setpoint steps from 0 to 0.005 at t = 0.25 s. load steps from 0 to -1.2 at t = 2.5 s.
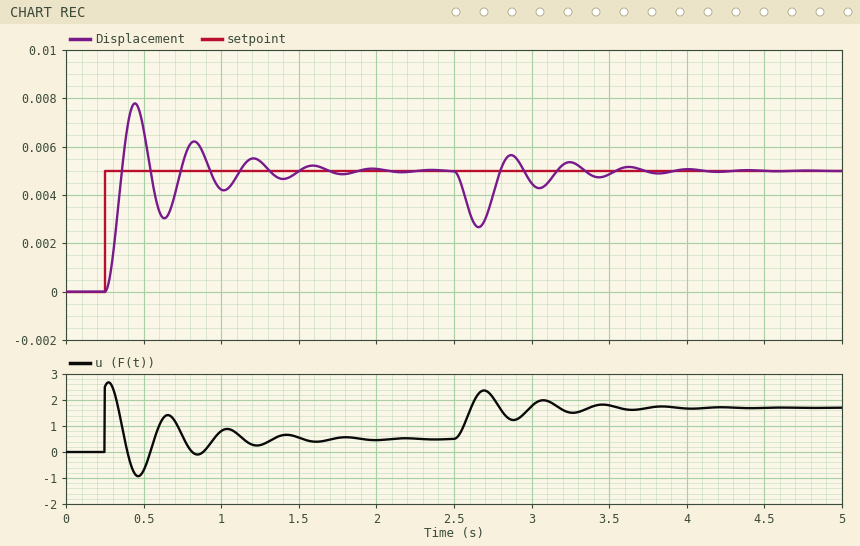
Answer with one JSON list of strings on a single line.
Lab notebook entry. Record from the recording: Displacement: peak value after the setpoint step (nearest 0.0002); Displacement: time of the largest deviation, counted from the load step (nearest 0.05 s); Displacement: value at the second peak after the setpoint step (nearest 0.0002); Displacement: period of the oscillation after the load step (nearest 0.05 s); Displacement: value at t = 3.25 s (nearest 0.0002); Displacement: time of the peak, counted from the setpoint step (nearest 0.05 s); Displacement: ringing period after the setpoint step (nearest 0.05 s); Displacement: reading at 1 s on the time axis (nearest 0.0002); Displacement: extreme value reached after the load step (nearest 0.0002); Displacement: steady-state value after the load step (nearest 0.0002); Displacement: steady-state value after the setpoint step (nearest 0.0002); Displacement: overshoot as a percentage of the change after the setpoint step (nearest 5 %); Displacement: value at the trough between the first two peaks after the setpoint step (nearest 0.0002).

["0.0078", "0.15 s", "0.0062", "0.40 s", "0.0054", "0.20 s", "0.40 s", "0.0042", "0.0026", "0.0050", "0.0050", "55 %", "0.0030"]
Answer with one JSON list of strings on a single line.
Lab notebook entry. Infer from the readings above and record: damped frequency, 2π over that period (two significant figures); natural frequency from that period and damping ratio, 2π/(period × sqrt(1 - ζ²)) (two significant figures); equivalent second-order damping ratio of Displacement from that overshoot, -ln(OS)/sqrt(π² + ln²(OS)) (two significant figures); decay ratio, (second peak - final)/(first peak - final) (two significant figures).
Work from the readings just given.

["16 rad/s", "16 rad/s", "0.19", "0.43"]
